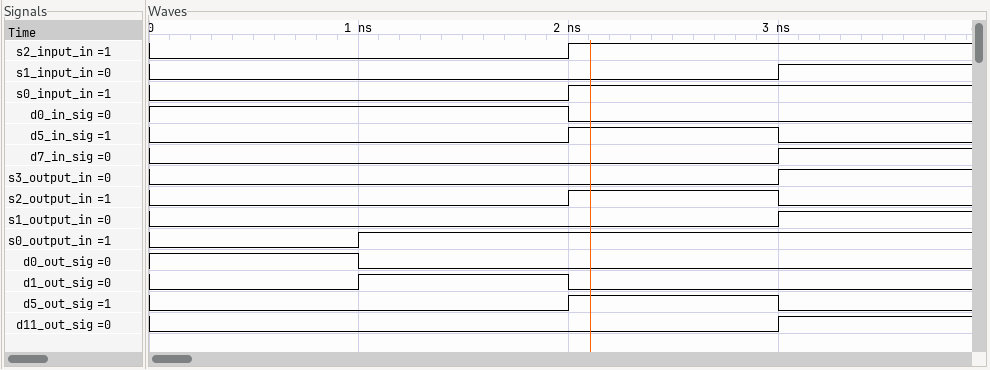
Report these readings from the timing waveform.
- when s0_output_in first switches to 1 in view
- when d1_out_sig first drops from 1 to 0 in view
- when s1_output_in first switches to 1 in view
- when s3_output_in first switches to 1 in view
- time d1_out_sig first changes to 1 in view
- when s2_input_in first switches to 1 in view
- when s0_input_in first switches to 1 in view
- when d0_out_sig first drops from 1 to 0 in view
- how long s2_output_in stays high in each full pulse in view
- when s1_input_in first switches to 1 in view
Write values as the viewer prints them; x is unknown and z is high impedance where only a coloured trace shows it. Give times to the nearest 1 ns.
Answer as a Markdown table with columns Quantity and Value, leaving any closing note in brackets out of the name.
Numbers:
| Quantity | Value |
|---|---|
| when s0_output_in first switches to 1 in view | 1 ns |
| when d1_out_sig first drops from 1 to 0 in view | 2 ns |
| when s1_output_in first switches to 1 in view | 3 ns |
| when s3_output_in first switches to 1 in view | 3 ns |
| time d1_out_sig first changes to 1 in view | 1 ns |
| when s2_input_in first switches to 1 in view | 2 ns |
| when s0_input_in first switches to 1 in view | 2 ns |
| when d0_out_sig first drops from 1 to 0 in view | 1 ns |
| how long s2_output_in stays high in each full pulse in view | 1 ns |
| when s1_input_in first switches to 1 in view | 3 ns |
